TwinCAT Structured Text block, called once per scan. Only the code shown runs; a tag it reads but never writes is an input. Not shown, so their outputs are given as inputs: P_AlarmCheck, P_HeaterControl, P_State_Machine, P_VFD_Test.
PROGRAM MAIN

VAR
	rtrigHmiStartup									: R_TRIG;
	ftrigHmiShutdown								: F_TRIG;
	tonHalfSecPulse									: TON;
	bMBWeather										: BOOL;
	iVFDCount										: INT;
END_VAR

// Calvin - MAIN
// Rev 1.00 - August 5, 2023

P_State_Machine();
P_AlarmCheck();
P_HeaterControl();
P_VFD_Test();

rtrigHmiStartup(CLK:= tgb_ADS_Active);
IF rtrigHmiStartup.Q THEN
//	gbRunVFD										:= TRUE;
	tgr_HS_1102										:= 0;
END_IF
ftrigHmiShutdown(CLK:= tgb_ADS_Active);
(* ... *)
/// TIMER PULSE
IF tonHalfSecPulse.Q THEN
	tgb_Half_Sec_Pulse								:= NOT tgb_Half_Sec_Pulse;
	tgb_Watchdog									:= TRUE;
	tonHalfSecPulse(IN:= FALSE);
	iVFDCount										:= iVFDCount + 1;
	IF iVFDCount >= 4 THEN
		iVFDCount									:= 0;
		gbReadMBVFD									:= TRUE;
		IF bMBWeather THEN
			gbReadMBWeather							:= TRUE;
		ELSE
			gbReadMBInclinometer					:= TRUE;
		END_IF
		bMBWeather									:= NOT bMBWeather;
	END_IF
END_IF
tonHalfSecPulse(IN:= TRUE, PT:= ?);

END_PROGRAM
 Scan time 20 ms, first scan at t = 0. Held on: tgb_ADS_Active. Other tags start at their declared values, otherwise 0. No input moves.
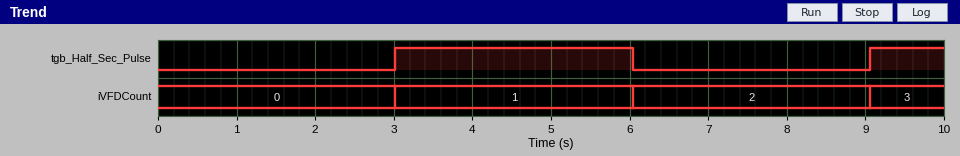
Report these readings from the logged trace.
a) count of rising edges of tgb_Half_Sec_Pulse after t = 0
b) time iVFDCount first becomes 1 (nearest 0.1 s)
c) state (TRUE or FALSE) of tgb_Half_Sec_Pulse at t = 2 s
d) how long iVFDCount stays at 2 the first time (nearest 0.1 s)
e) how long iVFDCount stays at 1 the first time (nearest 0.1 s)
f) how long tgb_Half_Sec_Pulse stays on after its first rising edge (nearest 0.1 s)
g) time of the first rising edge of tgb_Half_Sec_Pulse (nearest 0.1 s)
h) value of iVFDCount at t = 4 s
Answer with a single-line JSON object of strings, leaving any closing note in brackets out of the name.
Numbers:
{"count of rising edges of tgb_Half_Sec_Pulse after t = 0": "2", "time iVFDCount first becomes 1": "3.0 s", "state (TRUE or FALSE) of tgb_Half_Sec_Pulse at t = 2 s": "FALSE", "how long iVFDCount stays at 2 the first time": "3.0 s", "how long iVFDCount stays at 1 the first time": "3.0 s", "how long tgb_Half_Sec_Pulse stays on after its first rising edge": "3.0 s", "time of the first rising edge of tgb_Half_Sec_Pulse": "3.0 s", "value of iVFDCount at t = 4 s": "1"}
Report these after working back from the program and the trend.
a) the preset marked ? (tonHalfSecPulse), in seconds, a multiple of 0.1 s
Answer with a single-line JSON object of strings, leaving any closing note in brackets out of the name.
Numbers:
{"the preset marked ? (tonHalfSecPulse), in seconds, a multiple of 0.1 s": "3.0 s"}
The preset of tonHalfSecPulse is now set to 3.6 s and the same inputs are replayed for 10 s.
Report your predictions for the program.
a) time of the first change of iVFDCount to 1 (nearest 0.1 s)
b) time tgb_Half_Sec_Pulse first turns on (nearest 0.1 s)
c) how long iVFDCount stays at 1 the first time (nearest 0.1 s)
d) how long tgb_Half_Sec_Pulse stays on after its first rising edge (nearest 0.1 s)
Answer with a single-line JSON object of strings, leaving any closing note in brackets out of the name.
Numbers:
{"time of the first change of iVFDCount to 1": "3.6 s", "time tgb_Half_Sec_Pulse first turns on": "3.6 s", "how long iVFDCount stays at 1 the first time": "3.6 s", "how long tgb_Half_Sec_Pulse stays on after its first rising edge": "3.6 s"}
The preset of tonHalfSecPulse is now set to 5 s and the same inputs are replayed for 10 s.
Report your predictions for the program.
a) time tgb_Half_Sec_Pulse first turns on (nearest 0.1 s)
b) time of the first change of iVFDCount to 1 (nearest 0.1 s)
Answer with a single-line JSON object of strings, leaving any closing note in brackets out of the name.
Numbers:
{"time tgb_Half_Sec_Pulse first turns on": "5.0 s", "time of the first change of iVFDCount to 1": "5.0 s"}
